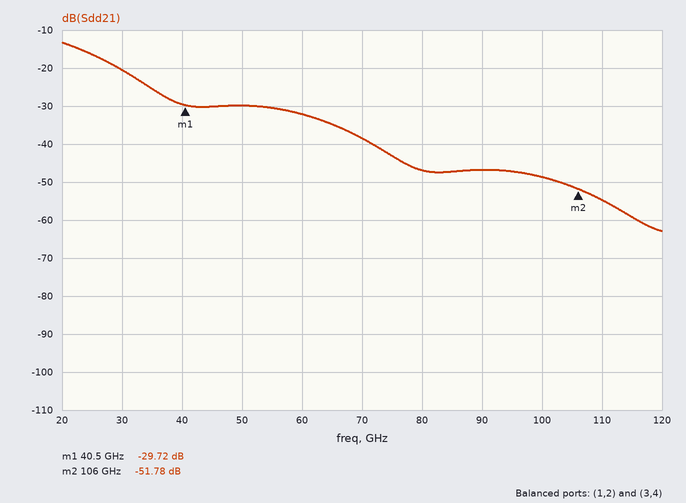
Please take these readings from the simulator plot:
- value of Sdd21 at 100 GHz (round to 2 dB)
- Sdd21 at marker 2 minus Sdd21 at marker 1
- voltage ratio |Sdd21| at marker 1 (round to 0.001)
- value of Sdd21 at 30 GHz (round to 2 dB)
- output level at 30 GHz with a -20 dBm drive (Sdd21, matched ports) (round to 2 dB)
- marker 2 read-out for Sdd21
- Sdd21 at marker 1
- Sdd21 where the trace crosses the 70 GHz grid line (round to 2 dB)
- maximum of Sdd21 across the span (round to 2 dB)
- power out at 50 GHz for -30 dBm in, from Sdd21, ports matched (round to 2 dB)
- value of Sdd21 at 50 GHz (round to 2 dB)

-48 dB
-22.06 dB
0.033
-20 dB
-40 dBm
-51.78 dB
-29.72 dB
-38 dB
-14 dB
-60 dBm
-30 dB
